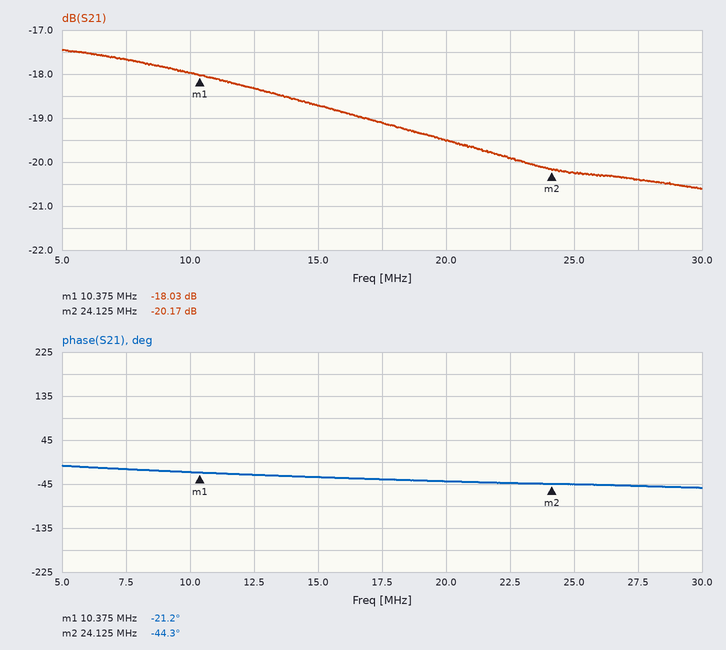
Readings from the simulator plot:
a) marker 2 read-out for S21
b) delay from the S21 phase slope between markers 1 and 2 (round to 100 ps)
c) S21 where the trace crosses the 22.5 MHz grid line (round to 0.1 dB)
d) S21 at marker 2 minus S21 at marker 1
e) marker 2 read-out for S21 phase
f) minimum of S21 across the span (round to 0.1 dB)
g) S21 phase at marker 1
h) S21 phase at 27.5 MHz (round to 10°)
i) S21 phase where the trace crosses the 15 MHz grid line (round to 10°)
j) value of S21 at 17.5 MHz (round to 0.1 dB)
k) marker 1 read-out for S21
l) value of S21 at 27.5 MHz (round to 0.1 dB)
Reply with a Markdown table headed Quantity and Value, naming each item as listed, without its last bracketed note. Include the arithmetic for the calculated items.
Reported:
| Quantity | Value |
|---|---|
| marker 2 read-out for S21 | -20.17 dB |
| delay from the S21 phase slope between markers 1 and 2 | −(-44.3° − (-21.2°))/(360° × 13.75 MHz) ≈ 4.7 ns |
| S21 where the trace crosses the 22.5 MHz grid line | -19.9 dB |
| S21 at marker 2 minus S21 at marker 1 | -20.17 − (-18.03) = -2.14 dB |
| marker 2 read-out for S21 phase | -44.3° |
| minimum of S21 across the span | -20.6 dB |
| S21 phase at marker 1 | -21.2° |
| S21 phase at 27.5 MHz | -50° |
| S21 phase where the trace crosses the 15 MHz grid line | -30° |
| value of S21 at 17.5 MHz | -19.1 dB |
| marker 1 read-out for S21 | -18.03 dB |
| value of S21 at 27.5 MHz | -20.4 dB |
